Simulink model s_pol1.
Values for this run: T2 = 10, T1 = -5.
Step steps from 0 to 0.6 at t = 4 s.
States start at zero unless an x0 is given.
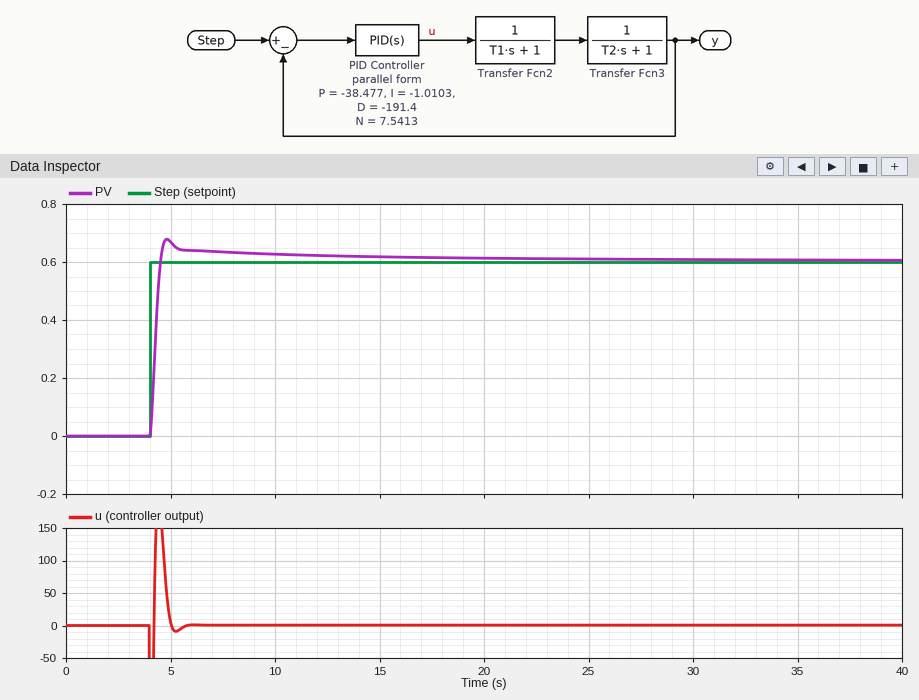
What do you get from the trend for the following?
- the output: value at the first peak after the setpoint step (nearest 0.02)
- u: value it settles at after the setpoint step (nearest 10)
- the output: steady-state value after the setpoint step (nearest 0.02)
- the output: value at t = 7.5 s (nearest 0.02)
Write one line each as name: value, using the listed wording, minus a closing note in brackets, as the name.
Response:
the output: value at the first peak after the setpoint step: 0.68
u: value it settles at after the setpoint step: 0
the output: steady-state value after the setpoint step: 0.60
the output: value at t = 7.5 s: 0.64
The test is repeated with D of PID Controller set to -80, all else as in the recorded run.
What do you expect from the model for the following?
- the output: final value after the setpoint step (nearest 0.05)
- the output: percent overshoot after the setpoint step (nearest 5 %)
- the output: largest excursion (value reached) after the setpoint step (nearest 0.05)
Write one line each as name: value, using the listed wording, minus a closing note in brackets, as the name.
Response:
the output: final value after the setpoint step: 0.60
the output: percent overshoot after the setpoint step: 25 %
the output: largest excursion (value reached) after the setpoint step: 0.75
